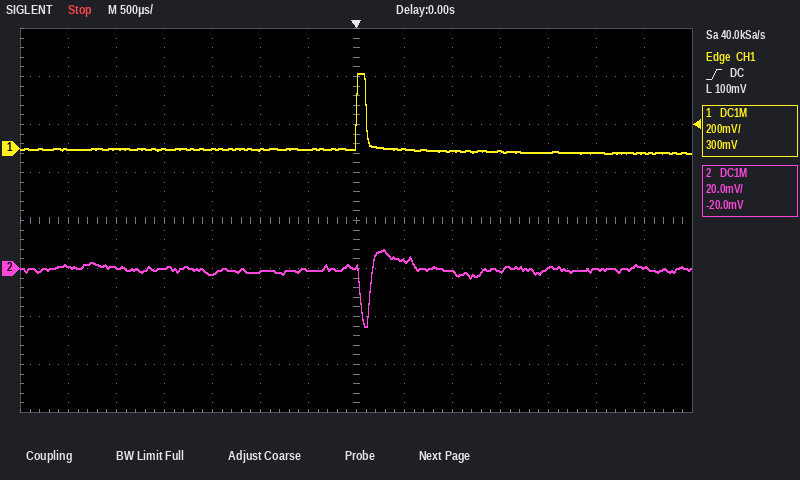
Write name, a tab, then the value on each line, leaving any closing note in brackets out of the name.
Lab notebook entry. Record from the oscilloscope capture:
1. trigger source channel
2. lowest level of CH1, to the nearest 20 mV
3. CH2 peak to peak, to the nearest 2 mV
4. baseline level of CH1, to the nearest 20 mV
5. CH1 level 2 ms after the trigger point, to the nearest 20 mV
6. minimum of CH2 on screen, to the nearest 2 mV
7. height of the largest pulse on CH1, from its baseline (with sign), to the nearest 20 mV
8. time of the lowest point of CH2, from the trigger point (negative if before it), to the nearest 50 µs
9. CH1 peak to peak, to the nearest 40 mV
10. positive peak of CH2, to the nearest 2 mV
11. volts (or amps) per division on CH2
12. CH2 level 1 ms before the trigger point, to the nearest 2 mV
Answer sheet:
trigger source channel	CH1
lowest level of CH1, to the nearest 20 mV	-20 mV
CH2 peak to peak, to the nearest 2 mV	32 mV
baseline level of CH1, to the nearest 20 mV	0 mV
CH1 level 2 ms after the trigger point, to the nearest 20 mV	-20 mV
minimum of CH2 on screen, to the nearest 2 mV	-24 mV
height of the largest pulse on CH1, from its baseline (with sign), to the nearest 20 mV	+320 mV
time of the lowest point of CH2, from the trigger point (negative if before it), to the nearest 50 µs	+100 µs
CH1 peak to peak, to the nearest 40 mV	320 mV
positive peak of CH2, to the nearest 2 mV	8 mV
volts (or amps) per division on CH2	20 mV
CH2 level 1 ms before the trigger point, to the nearest 2 mV	-2 mV
